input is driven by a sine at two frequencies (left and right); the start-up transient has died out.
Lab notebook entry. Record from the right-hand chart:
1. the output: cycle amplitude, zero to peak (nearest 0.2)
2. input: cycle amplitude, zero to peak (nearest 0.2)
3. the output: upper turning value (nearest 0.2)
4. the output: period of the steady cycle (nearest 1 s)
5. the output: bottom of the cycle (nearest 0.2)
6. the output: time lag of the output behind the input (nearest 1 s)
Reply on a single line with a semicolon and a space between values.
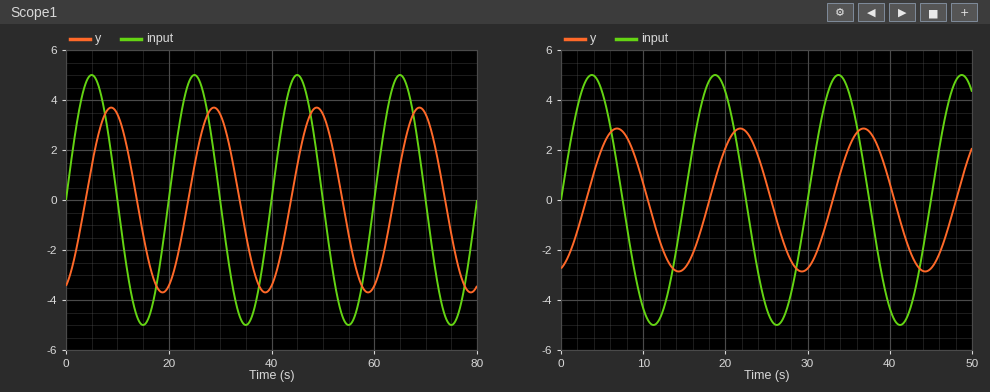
2.8; 5.0; 2.8; 15 s; -2.8; 3 s
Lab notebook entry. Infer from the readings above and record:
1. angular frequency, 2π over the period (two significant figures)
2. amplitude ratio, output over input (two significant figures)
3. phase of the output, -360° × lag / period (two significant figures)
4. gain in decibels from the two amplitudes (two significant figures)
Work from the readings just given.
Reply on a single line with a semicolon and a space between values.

0.42 rad/s; 0.56; -72°; -5.0 dB
